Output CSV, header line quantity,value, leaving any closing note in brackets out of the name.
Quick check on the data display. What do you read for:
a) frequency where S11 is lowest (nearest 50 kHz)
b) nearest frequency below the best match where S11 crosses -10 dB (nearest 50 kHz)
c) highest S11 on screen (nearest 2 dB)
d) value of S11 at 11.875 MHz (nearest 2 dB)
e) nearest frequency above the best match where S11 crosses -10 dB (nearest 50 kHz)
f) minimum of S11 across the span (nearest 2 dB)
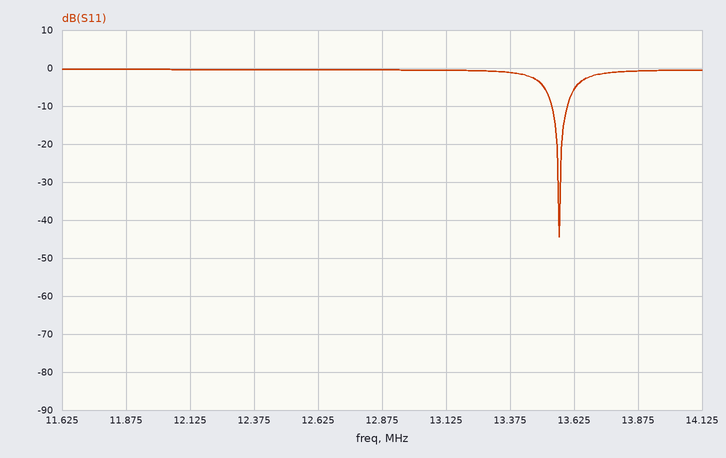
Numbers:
quantity,value
frequency where S11 is lowest,13.55 MHz
nearest frequency below the best match where S11 crosses -10 dB,13.55 MHz
highest S11 on screen,0 dB
value of S11 at 11.875 MHz,0 dB
nearest frequency above the best match where S11 crosses -10 dB,13.60 MHz
minimum of S11 across the span,-44 dB
